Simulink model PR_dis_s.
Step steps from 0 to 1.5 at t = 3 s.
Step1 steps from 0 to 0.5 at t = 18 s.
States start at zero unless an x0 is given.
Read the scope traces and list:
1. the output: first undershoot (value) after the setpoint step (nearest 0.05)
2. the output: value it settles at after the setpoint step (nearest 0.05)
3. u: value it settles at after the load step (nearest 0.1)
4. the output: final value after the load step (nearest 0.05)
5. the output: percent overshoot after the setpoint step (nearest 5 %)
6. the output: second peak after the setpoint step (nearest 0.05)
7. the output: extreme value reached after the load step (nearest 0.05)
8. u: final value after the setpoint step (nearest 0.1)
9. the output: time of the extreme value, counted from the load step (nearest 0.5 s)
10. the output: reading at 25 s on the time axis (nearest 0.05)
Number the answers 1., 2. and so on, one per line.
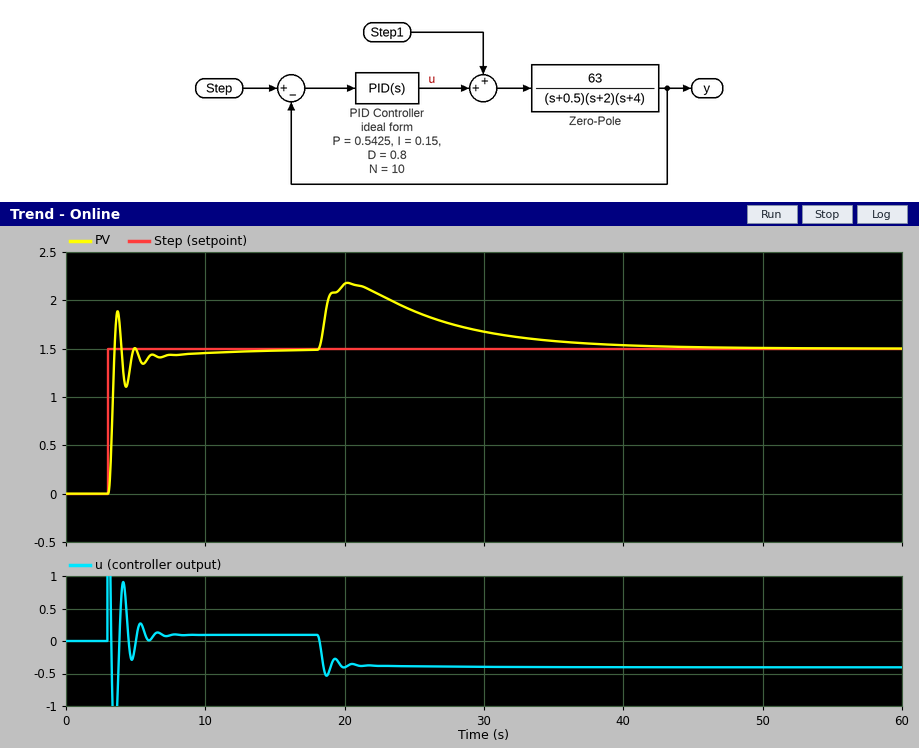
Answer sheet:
1. 1.10
2. 1.50
3. -0.4
4. 1.50
5. 25 %
6. 1.50
7. 2.20
8. 0.1
9. 2.0 s
10. 1.90
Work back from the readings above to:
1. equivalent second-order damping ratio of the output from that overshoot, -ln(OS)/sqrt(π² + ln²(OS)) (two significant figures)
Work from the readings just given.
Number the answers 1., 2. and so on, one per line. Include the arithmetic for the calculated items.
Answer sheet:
1. ln(0.25) = -1.386; 1.386 / sqrt(9.870 + 1.922) = 0.40
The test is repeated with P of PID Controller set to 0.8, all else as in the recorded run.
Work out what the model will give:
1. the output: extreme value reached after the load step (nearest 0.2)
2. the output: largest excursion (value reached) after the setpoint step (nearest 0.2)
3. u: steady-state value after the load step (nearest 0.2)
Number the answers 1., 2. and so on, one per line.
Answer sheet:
1. 2.0
2. 2.2
3. -0.4
